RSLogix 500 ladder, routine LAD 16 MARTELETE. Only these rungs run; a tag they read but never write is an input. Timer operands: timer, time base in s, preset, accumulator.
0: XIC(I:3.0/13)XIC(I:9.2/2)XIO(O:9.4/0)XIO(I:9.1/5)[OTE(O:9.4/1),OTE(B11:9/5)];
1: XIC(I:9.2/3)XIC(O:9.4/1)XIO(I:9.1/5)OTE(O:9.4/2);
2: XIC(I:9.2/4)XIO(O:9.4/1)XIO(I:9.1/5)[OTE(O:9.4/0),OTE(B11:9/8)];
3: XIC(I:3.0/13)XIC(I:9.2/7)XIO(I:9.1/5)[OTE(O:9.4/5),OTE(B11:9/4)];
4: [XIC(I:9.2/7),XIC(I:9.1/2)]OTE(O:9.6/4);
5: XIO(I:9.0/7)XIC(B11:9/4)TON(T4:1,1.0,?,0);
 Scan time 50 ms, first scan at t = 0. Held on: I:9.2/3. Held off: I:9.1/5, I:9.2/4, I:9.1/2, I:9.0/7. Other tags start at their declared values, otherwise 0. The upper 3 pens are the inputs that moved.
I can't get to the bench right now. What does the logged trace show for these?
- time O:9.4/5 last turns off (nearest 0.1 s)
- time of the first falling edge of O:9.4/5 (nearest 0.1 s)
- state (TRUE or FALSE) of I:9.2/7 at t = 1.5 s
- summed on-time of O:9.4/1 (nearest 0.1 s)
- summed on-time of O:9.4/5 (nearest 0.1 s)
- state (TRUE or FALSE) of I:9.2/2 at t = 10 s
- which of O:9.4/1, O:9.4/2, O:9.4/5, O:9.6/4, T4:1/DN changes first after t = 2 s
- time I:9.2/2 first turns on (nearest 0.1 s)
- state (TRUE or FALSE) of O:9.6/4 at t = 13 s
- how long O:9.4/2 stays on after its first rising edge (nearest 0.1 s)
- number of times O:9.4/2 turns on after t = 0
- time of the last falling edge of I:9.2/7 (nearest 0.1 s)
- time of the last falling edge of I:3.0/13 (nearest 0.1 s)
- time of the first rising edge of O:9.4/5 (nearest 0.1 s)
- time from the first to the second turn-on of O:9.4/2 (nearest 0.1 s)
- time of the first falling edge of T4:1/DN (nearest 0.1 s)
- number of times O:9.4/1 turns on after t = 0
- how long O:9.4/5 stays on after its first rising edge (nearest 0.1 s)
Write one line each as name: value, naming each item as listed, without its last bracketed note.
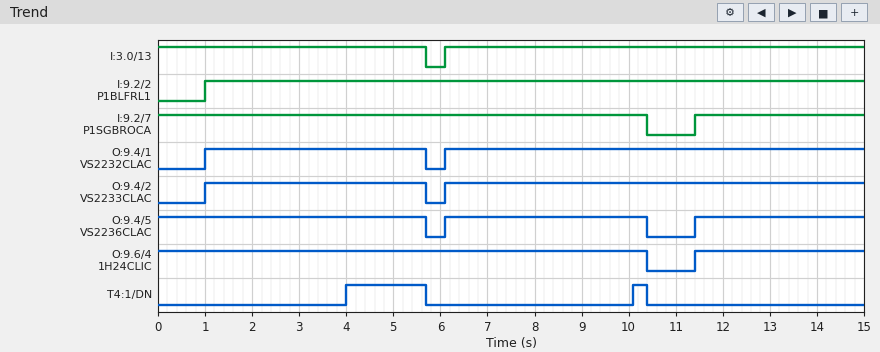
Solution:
time O:9.4/5 last turns off: 10.4 s
time of the first falling edge of O:9.4/5: 5.7 s
state (TRUE or FALSE) of I:9.2/7 at t = 1.5 s: TRUE
summed on-time of O:9.4/1: 13.6 s
summed on-time of O:9.4/5: 13.6 s
state (TRUE or FALSE) of I:9.2/2 at t = 10 s: TRUE
which of O:9.4/1, O:9.4/2, O:9.4/5, O:9.6/4, T4:1/DN changes first after t = 2 s: T4:1/DN
time I:9.2/2 first turns on: 1.0 s
state (TRUE or FALSE) of O:9.6/4 at t = 13 s: TRUE
how long O:9.4/2 stays on after its first rising edge: 4.7 s
number of times O:9.4/2 turns on after t = 0: 2
time of the last falling edge of I:9.2/7: 10.4 s
time of the last falling edge of I:3.0/13: 5.7 s
time of the first rising edge of O:9.4/5: 6.1 s
time from the first to the second turn-on of O:9.4/2: 5.1 s
time of the first falling edge of T4:1/DN: 5.7 s
number of times O:9.4/1 turns on after t = 0: 2
how long O:9.4/5 stays on after its first rising edge: 4.3 s
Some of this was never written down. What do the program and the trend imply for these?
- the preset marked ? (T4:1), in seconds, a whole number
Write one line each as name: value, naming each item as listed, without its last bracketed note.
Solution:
the preset marked ? (T4:1), in seconds, a whole number: 4 s
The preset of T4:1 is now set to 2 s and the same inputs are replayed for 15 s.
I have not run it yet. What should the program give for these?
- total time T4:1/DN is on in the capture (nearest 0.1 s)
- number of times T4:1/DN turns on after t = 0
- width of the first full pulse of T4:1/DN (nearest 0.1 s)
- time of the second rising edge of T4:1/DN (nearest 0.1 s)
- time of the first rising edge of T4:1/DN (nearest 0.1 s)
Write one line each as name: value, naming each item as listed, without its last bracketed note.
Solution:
total time T4:1/DN is on in the capture: 7.6 s
number of times T4:1/DN turns on after t = 0: 3
width of the first full pulse of T4:1/DN: 3.7 s
time of the second rising edge of T4:1/DN: 8.1 s
time of the first rising edge of T4:1/DN: 2.0 s
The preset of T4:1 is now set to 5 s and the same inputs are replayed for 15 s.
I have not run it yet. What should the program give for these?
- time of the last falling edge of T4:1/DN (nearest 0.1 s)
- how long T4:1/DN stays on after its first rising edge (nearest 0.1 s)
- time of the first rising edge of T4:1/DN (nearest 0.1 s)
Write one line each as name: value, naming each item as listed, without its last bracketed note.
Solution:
time of the last falling edge of T4:1/DN: 5.7 s
how long T4:1/DN stays on after its first rising edge: 0.7 s
time of the first rising edge of T4:1/DN: 5.0 s
